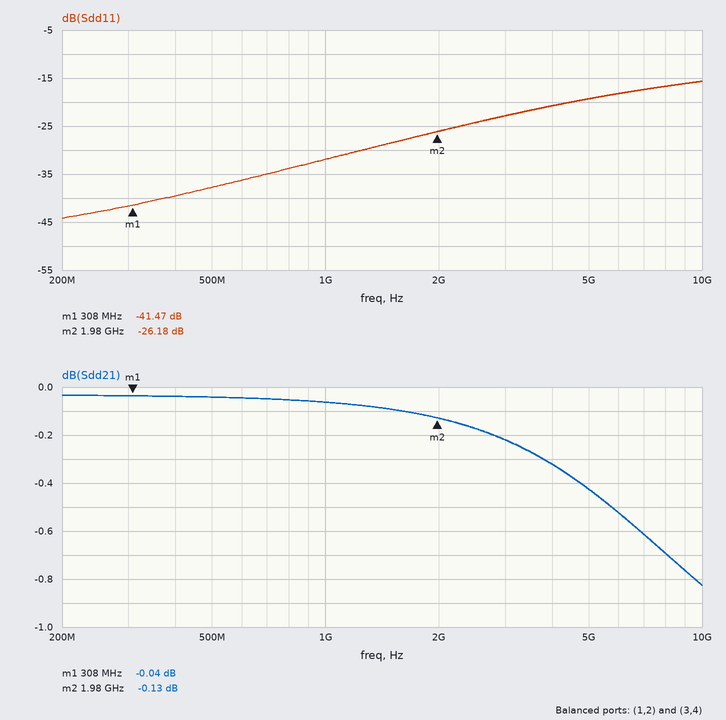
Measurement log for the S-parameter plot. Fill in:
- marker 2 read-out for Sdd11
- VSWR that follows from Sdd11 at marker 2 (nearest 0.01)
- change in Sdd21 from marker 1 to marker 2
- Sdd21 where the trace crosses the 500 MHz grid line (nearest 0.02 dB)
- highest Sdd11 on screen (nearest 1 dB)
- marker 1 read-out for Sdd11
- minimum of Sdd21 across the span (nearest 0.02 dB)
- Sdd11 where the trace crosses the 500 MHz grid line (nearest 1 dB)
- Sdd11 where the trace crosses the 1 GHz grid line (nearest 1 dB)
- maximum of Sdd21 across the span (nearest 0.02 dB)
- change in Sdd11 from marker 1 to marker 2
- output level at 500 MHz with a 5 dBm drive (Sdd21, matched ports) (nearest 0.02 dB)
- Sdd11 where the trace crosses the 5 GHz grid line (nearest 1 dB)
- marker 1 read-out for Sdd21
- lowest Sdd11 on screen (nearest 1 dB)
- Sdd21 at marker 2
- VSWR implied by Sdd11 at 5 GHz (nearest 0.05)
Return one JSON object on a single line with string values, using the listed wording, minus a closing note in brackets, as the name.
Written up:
{"marker 2 read-out for Sdd11": "-26.18 dB", "VSWR that follows from Sdd11 at marker 2": "1.10", "change in Sdd21 from marker 1 to marker 2": "-0.09 dB", "Sdd21 where the trace crosses the 500 MHz grid line": "-0.04 dB", "highest Sdd11 on screen": "-16 dB", "marker 1 read-out for Sdd11": "-41.47 dB", "minimum of Sdd21 across the span": "-0.82 dB", "Sdd11 where the trace crosses the 500 MHz grid line": "-38 dB", "Sdd11 where the trace crosses the 1 GHz grid line": "-32 dB", "maximum of Sdd21 across the span": "-0.04 dB", "change in Sdd11 from marker 1 to marker 2": "15.29 dB", "output level at 500 MHz with a 5 dBm drive (Sdd21, matched ports)": "4.96 dBm", "Sdd11 where the trace crosses the 5 GHz grid line": "-19 dB", "marker 1 read-out for Sdd21": "-0.04 dB", "lowest Sdd11 on screen": "-44 dB", "Sdd21 at marker 2": "-0.13 dB", "VSWR implied by Sdd11 at 5 GHz": "1.25"}
